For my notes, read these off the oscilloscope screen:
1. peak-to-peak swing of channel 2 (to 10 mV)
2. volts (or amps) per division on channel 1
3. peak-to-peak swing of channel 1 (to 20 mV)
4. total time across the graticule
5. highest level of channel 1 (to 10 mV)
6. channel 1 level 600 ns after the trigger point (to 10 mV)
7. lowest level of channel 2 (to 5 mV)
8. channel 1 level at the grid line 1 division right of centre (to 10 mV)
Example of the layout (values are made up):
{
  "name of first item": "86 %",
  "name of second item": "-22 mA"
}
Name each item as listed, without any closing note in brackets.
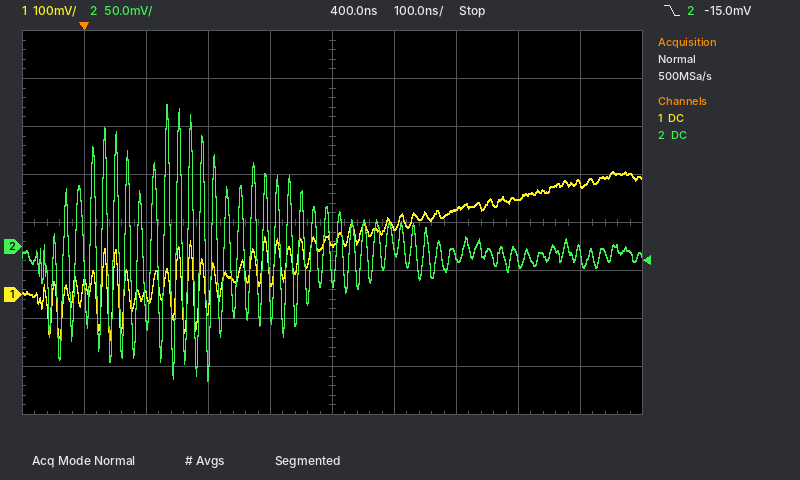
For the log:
{
  "peak-to-peak swing of channel 2": "290 mV",
  "volts (or amps) per division on channel 1": "100 mV",
  "peak-to-peak swing of channel 1": "360 mV",
  "total time across the graticule": "1 µs",
  "highest level of channel 1": "260 mV",
  "channel 1 level 600 ns after the trigger point": "180 mV",
  "lowest level of channel 2": "-140 mV",
  "channel 1 level at the grid line 1 division right of centre": "140 mV"
}
